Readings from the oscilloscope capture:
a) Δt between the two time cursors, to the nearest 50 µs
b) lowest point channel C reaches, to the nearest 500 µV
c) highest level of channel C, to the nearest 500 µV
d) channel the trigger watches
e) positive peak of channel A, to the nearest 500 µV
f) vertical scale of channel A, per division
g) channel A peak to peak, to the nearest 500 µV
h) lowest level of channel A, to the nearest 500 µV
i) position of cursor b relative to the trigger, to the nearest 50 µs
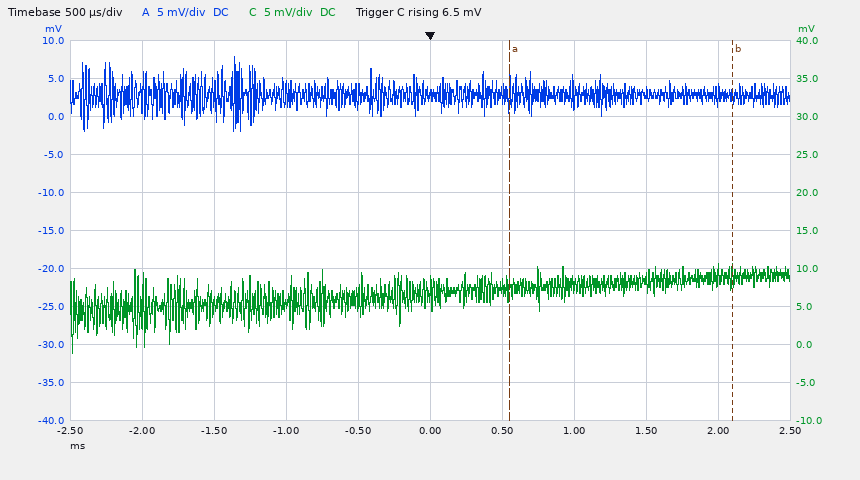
1.55 ms
-1.0 mV
10.5 mV
channel C
8.0 mV
5 mV
10.0 mV
-2.0 mV
+2.10 ms
